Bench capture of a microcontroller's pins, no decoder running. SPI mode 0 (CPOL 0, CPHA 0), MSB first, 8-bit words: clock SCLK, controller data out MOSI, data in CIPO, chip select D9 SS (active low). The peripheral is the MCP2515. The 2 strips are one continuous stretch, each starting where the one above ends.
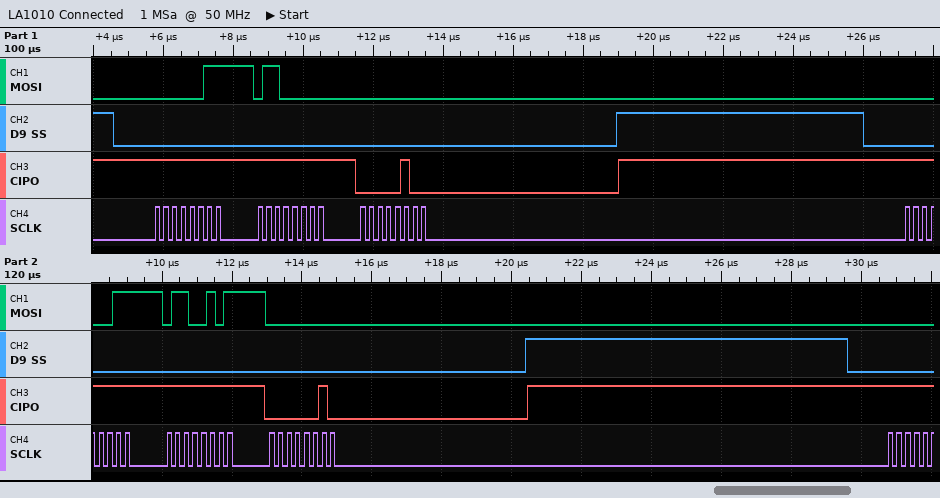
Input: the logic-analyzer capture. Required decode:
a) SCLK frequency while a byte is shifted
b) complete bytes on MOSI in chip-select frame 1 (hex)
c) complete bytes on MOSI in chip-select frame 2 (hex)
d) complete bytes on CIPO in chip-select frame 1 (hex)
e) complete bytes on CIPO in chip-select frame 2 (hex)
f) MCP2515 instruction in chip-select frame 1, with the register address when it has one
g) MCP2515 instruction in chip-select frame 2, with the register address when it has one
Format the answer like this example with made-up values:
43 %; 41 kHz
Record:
4 MHz; 0x03 0x60 0x00; 0x03 0x65 0x00; 0xFF 0xFF 0x04; 0xFF 0xFF 0x02; READ 0x60; READ 0x65
